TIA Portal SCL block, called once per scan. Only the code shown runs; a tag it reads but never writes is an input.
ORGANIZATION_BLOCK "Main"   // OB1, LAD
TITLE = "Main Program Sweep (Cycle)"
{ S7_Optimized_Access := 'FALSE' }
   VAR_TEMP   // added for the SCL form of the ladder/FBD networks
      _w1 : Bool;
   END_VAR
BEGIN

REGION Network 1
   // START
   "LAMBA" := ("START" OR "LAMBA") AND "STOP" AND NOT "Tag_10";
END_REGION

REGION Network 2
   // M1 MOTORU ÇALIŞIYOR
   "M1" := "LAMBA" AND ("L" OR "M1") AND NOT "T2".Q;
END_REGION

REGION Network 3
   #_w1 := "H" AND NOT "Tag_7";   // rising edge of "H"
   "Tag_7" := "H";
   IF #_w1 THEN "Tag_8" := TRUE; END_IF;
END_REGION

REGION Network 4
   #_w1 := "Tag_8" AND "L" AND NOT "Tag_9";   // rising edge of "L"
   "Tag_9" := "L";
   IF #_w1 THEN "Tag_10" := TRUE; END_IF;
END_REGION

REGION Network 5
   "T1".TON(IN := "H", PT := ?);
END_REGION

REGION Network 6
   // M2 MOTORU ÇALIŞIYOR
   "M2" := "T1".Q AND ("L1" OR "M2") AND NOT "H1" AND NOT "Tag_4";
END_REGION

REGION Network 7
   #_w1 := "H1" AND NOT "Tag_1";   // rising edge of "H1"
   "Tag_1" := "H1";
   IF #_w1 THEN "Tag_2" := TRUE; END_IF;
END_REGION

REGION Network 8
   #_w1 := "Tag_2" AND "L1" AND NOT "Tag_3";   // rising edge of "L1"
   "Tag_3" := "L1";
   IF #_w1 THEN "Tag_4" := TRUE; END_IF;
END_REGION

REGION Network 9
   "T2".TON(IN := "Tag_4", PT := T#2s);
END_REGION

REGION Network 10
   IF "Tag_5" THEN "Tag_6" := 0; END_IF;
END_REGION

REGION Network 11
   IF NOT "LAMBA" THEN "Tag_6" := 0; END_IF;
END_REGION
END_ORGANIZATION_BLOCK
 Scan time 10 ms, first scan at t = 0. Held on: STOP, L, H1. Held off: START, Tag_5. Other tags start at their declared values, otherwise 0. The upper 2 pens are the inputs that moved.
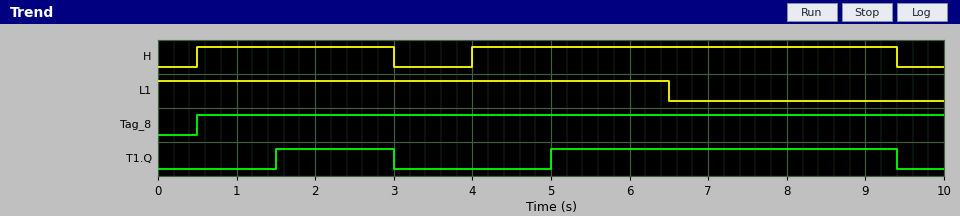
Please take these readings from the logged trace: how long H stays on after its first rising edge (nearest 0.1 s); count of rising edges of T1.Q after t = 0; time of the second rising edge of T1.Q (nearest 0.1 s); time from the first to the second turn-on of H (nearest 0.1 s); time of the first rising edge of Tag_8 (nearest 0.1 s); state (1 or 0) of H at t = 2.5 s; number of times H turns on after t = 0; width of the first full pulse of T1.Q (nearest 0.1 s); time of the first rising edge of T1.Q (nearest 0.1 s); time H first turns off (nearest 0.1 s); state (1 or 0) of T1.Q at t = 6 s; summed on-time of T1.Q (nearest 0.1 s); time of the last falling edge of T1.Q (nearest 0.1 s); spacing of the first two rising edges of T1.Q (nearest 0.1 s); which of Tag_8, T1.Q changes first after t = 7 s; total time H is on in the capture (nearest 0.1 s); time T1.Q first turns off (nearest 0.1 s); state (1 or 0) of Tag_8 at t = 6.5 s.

2.5 s
2
5.0 s
3.5 s
0.5 s
1
2
1.5 s
1.5 s
3.0 s
1
5.9 s
9.4 s
3.5 s
T1.Q
7.9 s
3.0 s
1
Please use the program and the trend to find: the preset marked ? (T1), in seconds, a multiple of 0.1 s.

1.0 s
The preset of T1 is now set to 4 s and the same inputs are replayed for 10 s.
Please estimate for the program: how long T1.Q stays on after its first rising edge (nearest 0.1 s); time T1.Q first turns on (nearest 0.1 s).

1.4 s
8.0 s
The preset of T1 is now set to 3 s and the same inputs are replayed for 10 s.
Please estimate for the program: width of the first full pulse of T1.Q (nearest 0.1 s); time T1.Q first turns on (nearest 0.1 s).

2.4 s
7.0 s
